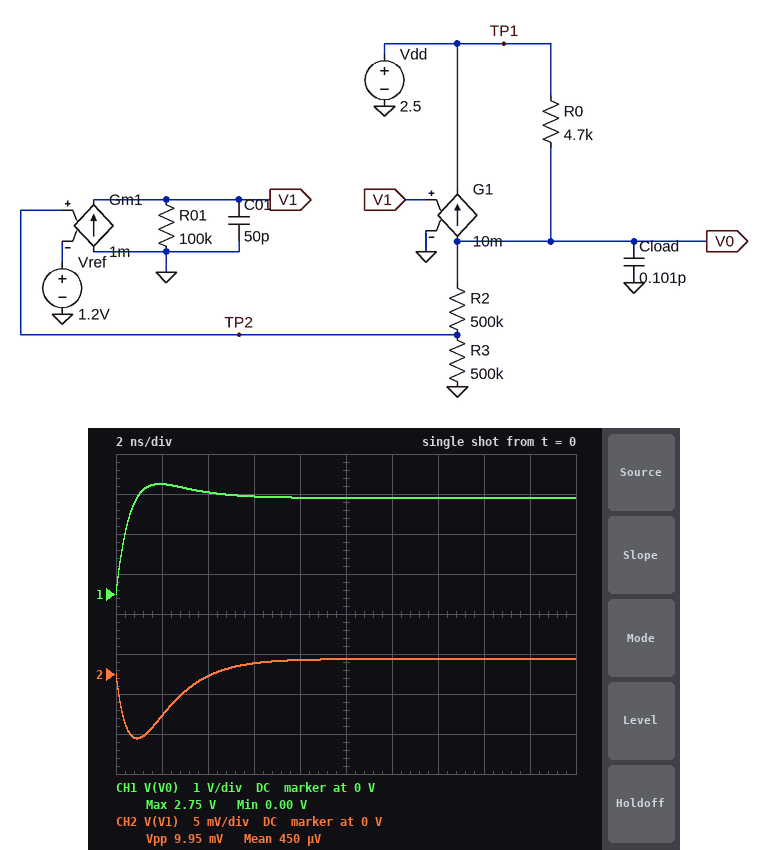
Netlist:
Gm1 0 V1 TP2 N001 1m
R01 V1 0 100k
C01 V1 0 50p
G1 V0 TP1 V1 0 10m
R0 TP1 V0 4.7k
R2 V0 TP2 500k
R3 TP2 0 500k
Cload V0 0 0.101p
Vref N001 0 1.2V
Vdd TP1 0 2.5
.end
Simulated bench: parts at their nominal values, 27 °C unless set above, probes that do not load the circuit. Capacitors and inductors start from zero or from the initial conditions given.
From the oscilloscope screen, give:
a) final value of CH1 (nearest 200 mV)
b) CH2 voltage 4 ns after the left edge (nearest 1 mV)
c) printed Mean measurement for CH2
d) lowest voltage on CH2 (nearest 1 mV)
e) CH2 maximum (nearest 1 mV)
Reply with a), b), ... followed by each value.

a) 2.4 V
b) 0 V
c) 450 µV
d) -8 mV
e) 2 mV
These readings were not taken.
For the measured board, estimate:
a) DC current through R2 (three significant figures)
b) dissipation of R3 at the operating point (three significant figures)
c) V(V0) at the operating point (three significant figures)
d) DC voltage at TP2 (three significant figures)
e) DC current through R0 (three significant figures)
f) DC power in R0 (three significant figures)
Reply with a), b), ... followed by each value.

a) 2.40 µA
b) 2.88 µW
c) 2.40 V
d) 1.20 V
e) 21.3 µA
f) 2.13 µW
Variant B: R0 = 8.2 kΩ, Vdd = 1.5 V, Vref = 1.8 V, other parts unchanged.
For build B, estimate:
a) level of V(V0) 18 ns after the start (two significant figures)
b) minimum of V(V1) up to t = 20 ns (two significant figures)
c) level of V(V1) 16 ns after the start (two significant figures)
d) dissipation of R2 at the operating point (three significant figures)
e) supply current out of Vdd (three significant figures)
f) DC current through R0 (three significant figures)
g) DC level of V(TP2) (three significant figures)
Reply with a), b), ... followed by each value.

a) 3.6 V
b) -34 mV
c) -26 mV
d) 6.48 µW
e) 3.60 µA
f) 256 µA
g) 1.80 V
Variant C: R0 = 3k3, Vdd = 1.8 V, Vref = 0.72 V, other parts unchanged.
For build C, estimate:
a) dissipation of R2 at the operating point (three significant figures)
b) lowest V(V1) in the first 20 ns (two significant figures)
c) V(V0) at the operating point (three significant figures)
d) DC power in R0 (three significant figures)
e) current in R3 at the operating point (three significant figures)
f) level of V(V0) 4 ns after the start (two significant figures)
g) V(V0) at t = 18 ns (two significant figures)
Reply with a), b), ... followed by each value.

a) 1.04 µW
b) -2.7 mV
c) 1.44 V
d) 39.2 µW
e) 1.44 µA
f) 1.6 V
g) 1.4 V
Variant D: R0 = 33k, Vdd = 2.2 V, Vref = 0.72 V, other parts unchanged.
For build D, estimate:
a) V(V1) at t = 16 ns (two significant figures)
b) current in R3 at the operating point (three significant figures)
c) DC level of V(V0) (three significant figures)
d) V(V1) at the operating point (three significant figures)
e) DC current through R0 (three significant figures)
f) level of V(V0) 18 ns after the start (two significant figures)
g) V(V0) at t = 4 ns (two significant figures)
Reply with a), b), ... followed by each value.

a) 2.4 mV
b) 1.44 µA
c) 1.44 V
d) 2.16 mV
e) 23.0 µA
f) 1.4 V
g) 1.8 V
